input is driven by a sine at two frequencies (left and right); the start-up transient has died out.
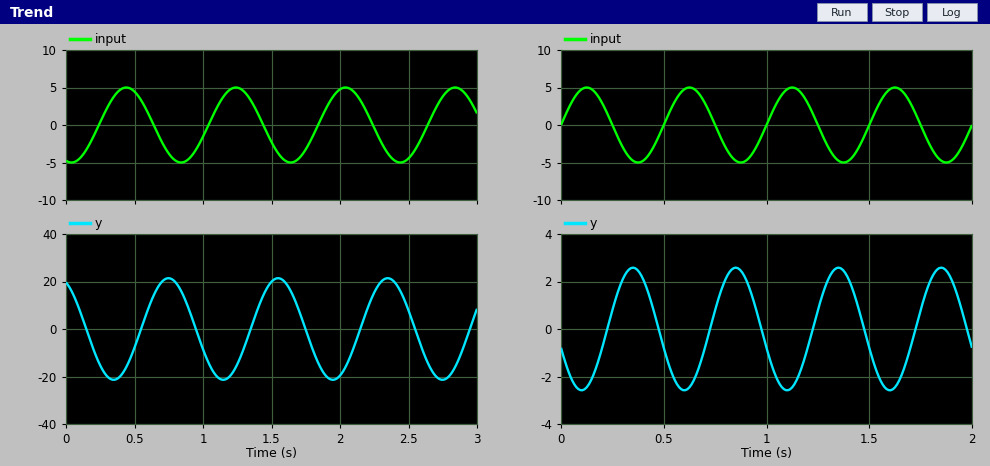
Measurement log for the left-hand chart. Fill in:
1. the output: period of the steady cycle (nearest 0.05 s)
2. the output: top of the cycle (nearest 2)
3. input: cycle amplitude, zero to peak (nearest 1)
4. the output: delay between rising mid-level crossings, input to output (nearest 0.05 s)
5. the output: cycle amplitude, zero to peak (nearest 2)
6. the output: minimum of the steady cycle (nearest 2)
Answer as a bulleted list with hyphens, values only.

- 0.80 s
- 22
- 5
- 0.30 s
- 22
- -22
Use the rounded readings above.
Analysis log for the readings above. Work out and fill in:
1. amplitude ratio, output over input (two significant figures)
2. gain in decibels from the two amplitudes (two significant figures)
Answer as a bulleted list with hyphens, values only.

- 4.4
- 13 dB
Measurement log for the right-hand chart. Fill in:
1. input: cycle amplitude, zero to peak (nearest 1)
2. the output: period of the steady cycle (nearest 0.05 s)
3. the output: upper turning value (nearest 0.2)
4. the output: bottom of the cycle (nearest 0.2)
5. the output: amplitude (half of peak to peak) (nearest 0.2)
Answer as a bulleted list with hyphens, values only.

- 5
- 0.50 s
- 2.6
- -2.6
- 2.6
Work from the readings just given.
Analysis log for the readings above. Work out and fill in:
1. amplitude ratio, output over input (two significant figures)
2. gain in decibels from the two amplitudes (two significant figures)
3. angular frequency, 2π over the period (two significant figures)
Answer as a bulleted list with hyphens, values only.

- 0.52
- -5.7 dB
- 13 rad/s
